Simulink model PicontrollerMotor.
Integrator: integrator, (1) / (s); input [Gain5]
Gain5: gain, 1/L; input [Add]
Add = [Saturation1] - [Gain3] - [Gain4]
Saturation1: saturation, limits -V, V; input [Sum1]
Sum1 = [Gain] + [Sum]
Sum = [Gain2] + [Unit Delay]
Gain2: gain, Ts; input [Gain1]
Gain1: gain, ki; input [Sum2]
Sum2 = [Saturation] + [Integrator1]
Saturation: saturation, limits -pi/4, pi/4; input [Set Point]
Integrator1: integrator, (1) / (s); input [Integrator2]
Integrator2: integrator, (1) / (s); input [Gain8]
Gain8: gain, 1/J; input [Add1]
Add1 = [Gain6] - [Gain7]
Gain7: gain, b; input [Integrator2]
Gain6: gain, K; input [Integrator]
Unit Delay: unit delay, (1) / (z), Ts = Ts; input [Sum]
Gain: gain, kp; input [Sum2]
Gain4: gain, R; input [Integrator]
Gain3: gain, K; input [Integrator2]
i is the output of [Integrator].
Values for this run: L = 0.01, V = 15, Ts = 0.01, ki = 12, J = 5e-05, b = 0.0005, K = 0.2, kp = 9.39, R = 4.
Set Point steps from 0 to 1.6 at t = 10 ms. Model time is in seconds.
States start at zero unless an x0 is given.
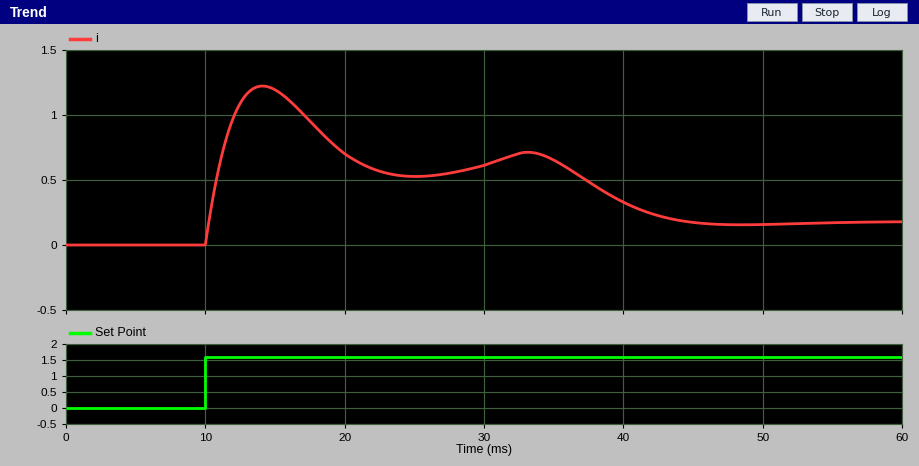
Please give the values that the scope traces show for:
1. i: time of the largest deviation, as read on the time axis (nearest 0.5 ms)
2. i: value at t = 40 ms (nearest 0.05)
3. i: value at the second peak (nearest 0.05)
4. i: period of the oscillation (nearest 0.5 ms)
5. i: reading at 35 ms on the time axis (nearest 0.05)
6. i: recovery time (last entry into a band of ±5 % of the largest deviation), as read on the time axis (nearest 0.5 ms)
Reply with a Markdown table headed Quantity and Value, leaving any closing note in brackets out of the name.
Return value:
| Quantity | Value |
|---|---|
| i: time of the largest deviation, as read on the time axis | 14.0 ms |
| i: value at t = 40 ms | 0.35 |
| i: value at the second peak | 0.70 |
| i: period of the oscillation | 19.0 ms |
| i: reading at 35 ms on the time axis | 0.65 |
| i: recovery time (last entry into a band of ±5 % of the largest deviation), as read on the time axis | 42.0 ms |
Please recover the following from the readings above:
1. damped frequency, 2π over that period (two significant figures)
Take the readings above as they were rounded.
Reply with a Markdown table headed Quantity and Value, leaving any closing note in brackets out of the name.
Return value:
| Quantity | Value |
|---|---|
| damped frequency, 2π over that period | 0.33 rad/ms |
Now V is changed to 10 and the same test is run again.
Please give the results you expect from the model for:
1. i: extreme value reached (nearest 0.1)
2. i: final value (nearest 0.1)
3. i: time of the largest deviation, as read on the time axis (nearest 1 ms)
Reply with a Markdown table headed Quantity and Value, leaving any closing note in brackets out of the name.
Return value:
| Quantity | Value |
|---|---|
| i: extreme value reached | 1.2 |
| i: final value | 0.1 |
| i: time of the largest deviation, as read on the time axis | 14 ms |
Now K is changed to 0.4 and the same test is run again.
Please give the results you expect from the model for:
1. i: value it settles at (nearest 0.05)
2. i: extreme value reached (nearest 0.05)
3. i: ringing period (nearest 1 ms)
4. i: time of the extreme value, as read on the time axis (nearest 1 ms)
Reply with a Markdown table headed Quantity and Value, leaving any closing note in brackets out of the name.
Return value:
| Quantity | Value |
|---|---|
| i: value it settles at | 0.05 |
| i: extreme value reached | 0.85 |
| i: ringing period | 12 ms |
| i: time of the extreme value, as read on the time axis | 12 ms |
